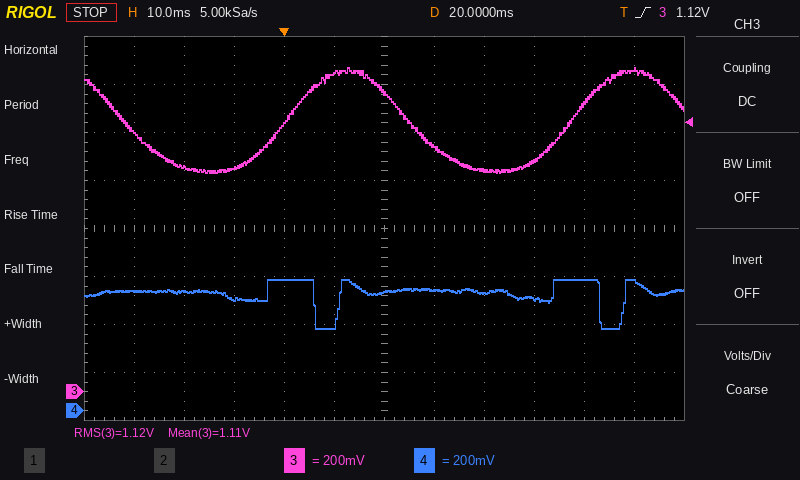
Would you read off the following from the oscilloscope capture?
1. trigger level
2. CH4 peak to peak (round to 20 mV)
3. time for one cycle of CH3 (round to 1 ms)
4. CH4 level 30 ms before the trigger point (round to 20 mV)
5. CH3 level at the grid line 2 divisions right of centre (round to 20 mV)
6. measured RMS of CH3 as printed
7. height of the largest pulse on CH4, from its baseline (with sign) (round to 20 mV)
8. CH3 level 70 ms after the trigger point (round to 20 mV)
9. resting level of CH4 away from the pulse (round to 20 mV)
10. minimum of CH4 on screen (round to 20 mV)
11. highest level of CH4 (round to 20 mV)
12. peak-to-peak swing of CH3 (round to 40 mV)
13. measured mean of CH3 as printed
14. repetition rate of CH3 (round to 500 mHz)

1.12 V
200 mV
57 ms
500 mV
920 mV
1.12 V
-160 mV
1.34 V
500 mV
340 mV
540 mV
440 mV
1.11 V
17.5 Hz
